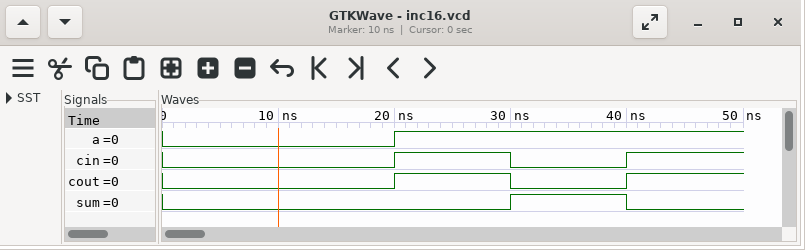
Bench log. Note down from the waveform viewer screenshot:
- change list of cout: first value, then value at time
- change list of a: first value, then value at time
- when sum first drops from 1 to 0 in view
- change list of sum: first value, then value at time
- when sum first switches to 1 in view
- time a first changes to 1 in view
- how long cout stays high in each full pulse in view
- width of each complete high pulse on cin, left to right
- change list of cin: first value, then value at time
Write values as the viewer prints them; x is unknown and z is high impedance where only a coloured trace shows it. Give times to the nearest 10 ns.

0, 1 at 20 ns, 0 at 30 ns, 1 at 40 ns
0, 1 at 20 ns
40 ns
0, 1 at 30 ns, 0 at 40 ns
30 ns
20 ns
10 ns
10 ns
0, 1 at 20 ns, 0 at 30 ns, 1 at 40 ns
